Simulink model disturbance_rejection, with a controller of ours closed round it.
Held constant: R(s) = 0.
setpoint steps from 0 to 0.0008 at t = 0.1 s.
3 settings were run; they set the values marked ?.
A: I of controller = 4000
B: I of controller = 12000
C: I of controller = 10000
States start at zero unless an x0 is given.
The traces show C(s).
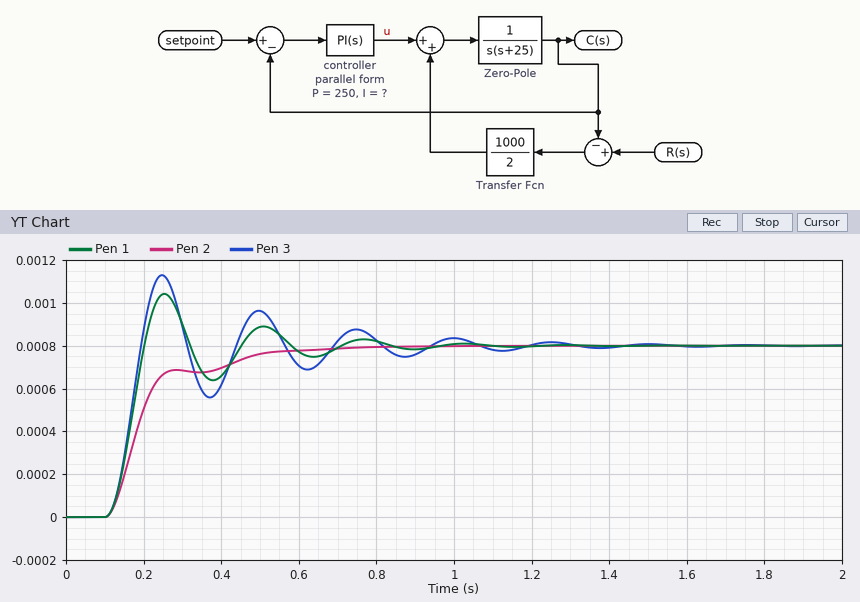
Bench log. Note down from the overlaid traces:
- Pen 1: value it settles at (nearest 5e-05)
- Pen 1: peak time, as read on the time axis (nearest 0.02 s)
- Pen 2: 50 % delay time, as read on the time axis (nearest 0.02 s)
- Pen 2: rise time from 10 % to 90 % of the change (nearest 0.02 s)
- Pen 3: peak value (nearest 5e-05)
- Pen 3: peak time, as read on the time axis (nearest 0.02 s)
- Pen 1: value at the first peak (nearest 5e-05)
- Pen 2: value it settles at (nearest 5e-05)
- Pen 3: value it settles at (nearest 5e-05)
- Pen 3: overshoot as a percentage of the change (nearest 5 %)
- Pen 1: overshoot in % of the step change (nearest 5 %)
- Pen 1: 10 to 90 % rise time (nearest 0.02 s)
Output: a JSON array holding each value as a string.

["0.00080", "0.26 s", "0.18 s", "0.30 s", "0.00115", "0.24 s", "0.00105", "0.00080", "0.00080", "40 %", "30 %", "0.06 s"]
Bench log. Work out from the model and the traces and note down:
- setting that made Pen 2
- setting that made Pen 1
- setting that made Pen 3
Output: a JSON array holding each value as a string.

["A", "C", "B"]
